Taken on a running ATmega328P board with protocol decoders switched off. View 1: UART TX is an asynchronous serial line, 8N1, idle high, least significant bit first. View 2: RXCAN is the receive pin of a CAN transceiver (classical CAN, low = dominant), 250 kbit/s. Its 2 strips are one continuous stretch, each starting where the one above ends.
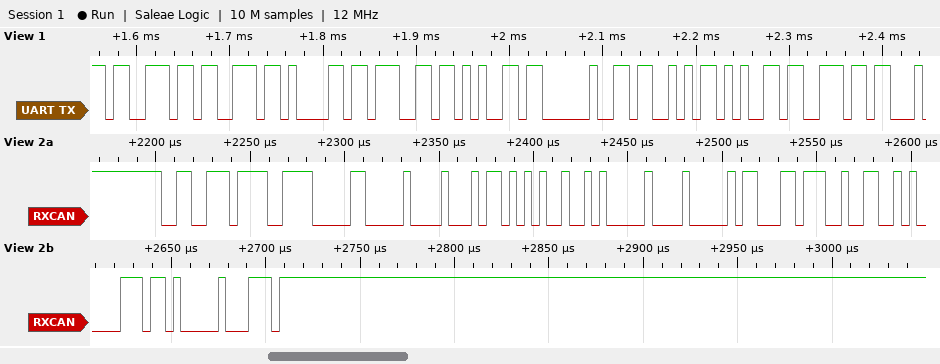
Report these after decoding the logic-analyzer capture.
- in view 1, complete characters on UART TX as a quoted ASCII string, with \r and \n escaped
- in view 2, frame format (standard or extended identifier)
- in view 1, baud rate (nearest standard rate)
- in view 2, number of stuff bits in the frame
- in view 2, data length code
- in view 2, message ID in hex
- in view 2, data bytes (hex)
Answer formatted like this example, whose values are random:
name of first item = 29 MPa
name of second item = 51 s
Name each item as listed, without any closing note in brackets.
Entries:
in view 1, complete characters on UART TX as a quoted ASCII string, with \r and \n escaped = "ssage Sen"
in view 2, frame format = extended
in view 1, baud rate = 115200 baud
in view 2, number of stuff bits in the frame = 6
in view 2, data length code = 8
in view 2, message ID in hex = 0x0CECF040
in view 2, data bytes = B5 49 40 10 31 B9 32 83
